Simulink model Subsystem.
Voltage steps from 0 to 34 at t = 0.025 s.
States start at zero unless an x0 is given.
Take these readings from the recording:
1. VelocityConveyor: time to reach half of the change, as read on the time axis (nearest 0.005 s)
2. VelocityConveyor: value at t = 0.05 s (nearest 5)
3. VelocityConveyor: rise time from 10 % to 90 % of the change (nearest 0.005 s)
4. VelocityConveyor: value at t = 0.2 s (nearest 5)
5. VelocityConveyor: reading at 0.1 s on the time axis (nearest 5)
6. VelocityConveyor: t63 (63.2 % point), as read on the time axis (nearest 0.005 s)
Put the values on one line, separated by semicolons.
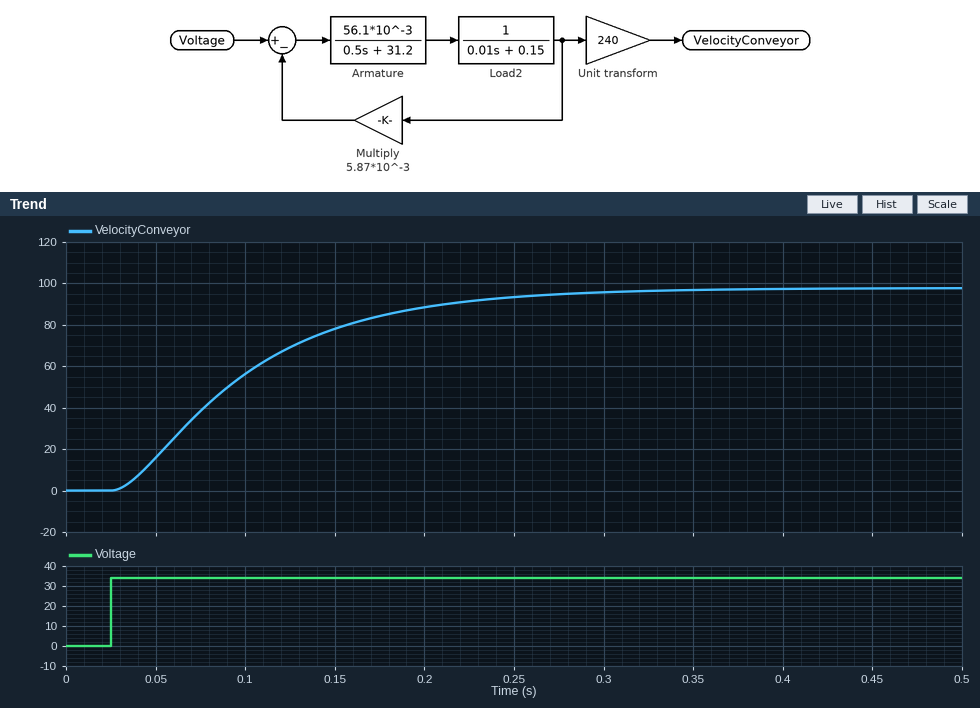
0.090 s; 15; 0.155 s; 90; 55; 0.110 s
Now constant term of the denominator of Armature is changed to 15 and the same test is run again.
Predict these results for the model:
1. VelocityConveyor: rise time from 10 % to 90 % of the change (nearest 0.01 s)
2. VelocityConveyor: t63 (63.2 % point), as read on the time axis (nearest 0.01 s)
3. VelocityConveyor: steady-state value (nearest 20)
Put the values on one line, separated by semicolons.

0.17 s; 0.13 s; 200
